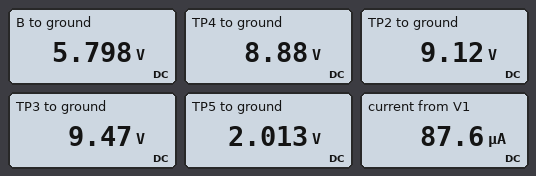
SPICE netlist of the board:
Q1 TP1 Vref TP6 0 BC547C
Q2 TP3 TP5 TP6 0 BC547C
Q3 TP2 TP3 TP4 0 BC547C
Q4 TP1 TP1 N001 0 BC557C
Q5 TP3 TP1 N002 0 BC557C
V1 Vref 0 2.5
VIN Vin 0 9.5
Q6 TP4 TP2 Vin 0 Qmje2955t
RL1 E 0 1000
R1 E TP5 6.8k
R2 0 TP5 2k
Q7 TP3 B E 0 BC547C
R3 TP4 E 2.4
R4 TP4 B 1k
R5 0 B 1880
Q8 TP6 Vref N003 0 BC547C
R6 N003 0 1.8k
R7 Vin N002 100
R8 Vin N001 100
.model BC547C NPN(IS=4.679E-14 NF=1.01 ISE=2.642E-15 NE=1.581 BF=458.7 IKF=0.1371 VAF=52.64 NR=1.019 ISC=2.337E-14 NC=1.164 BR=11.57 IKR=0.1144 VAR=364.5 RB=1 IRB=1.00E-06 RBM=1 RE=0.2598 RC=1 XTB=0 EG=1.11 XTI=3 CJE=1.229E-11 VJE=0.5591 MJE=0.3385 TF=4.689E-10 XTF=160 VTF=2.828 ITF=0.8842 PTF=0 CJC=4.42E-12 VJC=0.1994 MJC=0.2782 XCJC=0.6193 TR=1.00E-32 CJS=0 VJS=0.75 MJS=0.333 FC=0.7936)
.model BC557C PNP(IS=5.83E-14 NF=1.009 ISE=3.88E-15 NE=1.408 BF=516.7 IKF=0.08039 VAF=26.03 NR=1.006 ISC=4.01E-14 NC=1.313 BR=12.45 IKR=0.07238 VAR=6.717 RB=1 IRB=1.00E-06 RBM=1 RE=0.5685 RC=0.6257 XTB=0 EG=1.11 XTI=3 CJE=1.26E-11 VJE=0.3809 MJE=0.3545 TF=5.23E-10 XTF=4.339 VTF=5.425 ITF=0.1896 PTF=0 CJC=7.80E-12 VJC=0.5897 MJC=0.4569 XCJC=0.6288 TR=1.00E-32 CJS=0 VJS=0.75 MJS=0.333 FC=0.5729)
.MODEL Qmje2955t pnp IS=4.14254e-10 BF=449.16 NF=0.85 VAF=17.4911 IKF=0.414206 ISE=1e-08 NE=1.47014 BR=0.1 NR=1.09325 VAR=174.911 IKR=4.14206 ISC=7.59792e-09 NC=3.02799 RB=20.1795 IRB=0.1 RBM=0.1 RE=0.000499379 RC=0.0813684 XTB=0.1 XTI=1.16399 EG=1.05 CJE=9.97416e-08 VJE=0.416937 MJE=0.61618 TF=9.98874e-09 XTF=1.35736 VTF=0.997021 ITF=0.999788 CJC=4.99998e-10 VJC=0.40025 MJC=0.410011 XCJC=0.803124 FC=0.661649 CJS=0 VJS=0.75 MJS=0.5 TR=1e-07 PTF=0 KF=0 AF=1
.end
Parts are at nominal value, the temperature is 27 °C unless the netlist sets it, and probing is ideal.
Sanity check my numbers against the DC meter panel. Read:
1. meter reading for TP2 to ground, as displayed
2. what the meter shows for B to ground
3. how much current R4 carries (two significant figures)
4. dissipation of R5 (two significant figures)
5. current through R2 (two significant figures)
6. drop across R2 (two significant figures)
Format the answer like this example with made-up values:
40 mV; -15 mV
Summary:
9.12 V; 5.798 V; 3.1 mA; 18 mW; 1.0 mA; 2.0 V
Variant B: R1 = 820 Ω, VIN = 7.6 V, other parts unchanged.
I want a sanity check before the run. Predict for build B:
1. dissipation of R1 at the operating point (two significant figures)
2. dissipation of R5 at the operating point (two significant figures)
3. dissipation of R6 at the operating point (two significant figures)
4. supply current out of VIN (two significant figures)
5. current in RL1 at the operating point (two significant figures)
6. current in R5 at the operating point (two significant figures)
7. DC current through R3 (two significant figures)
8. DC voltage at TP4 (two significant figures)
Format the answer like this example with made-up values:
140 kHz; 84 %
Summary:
1.3 mW; 2.8 mW; 1.9 mW; 7.0 mA; 3.5 mA; 1.2 mA; 4.8 mA; 3.5 V
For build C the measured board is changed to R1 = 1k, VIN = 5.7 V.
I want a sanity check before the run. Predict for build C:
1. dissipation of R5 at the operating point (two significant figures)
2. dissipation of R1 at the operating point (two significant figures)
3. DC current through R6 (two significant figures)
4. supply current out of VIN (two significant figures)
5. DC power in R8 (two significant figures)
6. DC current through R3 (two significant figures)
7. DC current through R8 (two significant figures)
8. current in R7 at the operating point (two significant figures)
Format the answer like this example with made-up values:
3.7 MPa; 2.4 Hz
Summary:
3.2 mW; 1.6 mW; 1.0 mA; 7.3 mA; 24 µW; 5.0 mA; 490 µA; 500 µA
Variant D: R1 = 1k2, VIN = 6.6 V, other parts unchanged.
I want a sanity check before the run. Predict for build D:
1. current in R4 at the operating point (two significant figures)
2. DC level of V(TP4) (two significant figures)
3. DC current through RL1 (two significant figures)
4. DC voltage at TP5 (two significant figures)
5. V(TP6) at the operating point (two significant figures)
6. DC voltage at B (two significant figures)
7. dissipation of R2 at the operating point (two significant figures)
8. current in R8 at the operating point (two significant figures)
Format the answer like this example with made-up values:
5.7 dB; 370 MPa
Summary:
1.4 mA; 4.0 V; 4.0 mA; 2.5 V; 1.9 V; 2.6 V; 3.1 mW; 490 µA
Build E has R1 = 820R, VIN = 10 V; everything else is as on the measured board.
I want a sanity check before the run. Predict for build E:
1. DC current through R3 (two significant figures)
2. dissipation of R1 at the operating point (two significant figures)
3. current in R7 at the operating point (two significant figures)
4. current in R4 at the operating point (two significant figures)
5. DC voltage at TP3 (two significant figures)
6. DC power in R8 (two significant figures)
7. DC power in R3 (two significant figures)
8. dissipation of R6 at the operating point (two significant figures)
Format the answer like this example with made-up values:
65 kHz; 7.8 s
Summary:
4.8 mA; 1.3 mW; 510 µA; 1.2 mA; 4.1 V; 23 µW; 55 µW; 1.9 mW
